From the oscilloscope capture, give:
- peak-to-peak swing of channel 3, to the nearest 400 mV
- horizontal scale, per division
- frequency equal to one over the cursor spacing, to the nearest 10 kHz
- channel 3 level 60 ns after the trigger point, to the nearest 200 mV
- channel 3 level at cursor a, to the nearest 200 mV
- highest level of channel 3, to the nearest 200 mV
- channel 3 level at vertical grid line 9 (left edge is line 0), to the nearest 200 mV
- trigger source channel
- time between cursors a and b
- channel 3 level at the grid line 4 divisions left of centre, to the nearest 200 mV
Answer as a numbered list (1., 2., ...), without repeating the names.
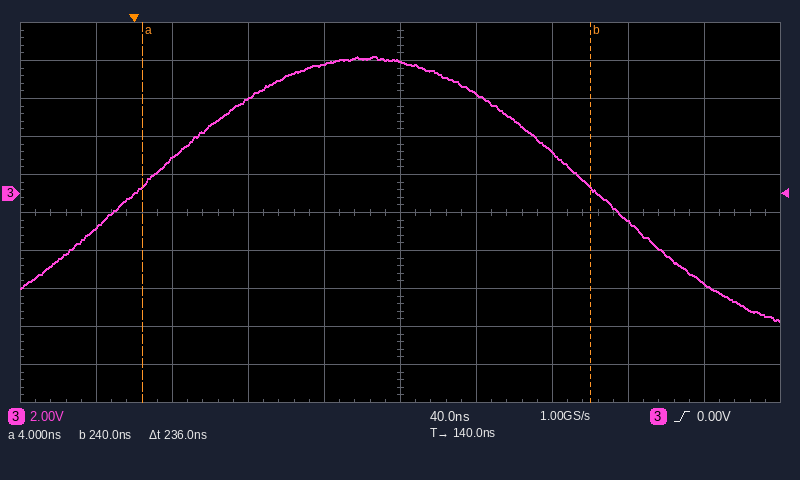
1. 14.0 V
2. 40 ns
3. 4.24 MHz
4. 5.0 V
5. 400 mV
6. 7.2 V
7. -4.8 V
8. channel 3
9. 236 ns
10. -1.8 V
